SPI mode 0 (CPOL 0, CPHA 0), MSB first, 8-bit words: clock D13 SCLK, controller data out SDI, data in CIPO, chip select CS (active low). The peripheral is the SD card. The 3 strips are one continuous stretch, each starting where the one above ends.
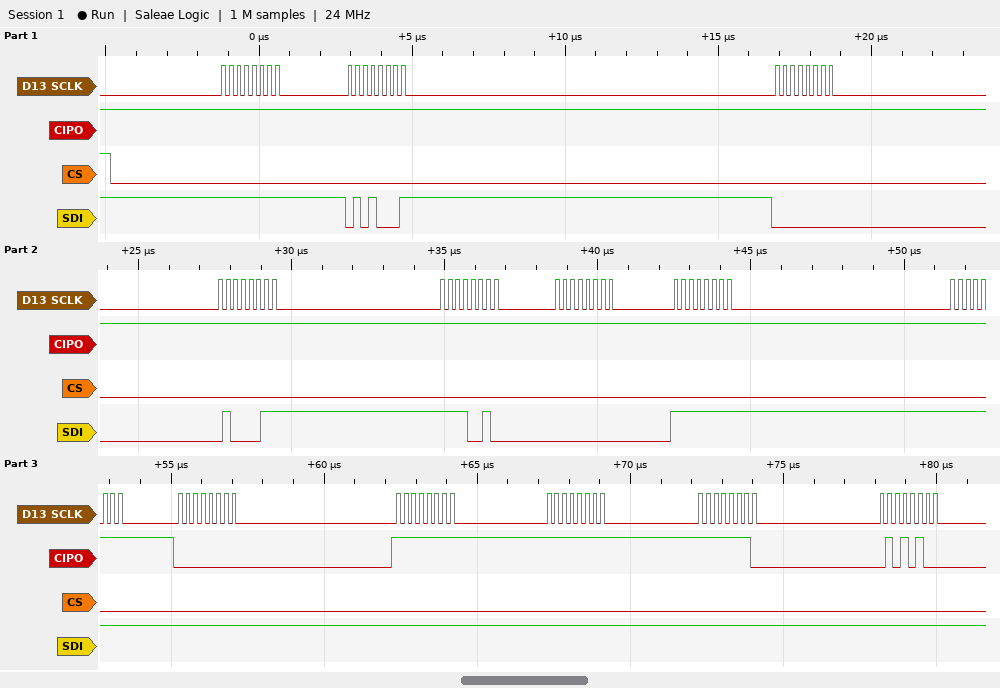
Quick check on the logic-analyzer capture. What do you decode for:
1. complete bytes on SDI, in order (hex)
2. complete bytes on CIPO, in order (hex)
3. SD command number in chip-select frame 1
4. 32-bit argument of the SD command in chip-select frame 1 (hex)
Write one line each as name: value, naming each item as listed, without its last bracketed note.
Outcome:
complete bytes on SDI, in order: FF 51 00 43 F2 00 FF FF FF FF FF FF FF
complete bytes on CIPO, in order: FF FF FF FF FF FF FF FF 00 FF FF FE 54
SD command number in chip-select frame 1: CMD17
32-bit argument of the SD command in chip-select frame 1: 0x0043F200
